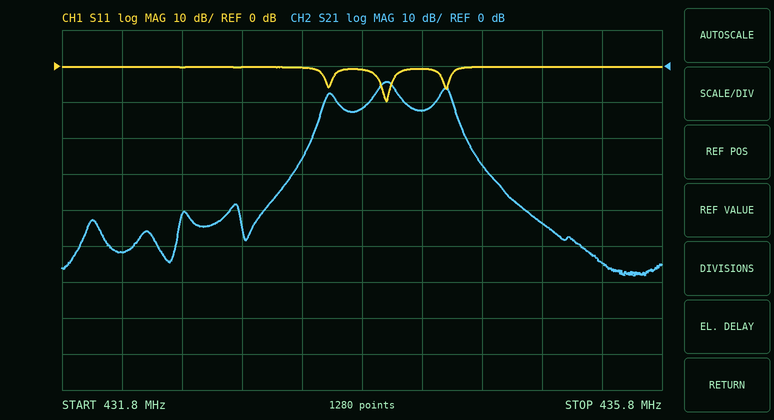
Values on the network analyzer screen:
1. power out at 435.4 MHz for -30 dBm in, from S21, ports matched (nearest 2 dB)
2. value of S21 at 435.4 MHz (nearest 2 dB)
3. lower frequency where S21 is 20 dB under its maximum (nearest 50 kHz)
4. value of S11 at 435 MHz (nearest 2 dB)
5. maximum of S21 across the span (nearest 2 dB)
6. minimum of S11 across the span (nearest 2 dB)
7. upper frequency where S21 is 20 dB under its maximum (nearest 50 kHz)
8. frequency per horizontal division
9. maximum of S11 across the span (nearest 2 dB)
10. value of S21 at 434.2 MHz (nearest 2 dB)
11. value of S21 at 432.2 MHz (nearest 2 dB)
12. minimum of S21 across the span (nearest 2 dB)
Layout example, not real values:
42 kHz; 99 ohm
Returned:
-84 dBm; -54 dB; 433.40 MHz; 0 dB; -4 dB; -10 dB; 434.55 MHz; 400 kHz; 0 dB; -12 dB; -52 dB; -58 dB
